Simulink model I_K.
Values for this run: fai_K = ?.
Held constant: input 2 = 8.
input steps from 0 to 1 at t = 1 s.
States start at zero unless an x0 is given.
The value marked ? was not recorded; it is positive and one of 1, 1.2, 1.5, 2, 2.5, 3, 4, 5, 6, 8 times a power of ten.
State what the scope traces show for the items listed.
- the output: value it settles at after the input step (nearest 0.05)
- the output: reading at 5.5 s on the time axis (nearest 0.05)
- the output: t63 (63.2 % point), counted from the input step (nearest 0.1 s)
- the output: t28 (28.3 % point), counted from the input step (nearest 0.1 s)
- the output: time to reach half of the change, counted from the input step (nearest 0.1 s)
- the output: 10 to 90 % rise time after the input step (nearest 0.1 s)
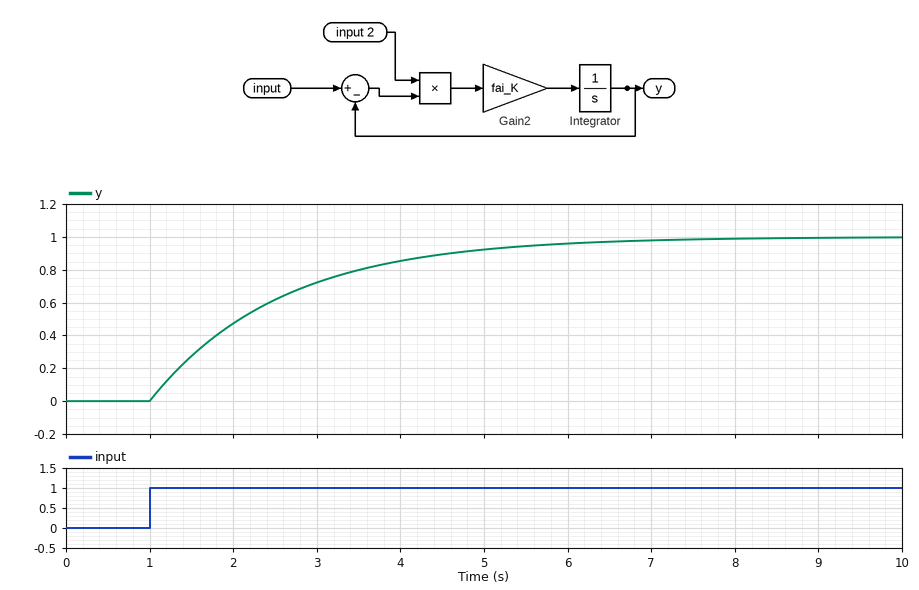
1.00
0.95
1.6 s
0.5 s
1.1 s
3.4 s
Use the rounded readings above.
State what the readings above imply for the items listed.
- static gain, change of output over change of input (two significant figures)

1.0
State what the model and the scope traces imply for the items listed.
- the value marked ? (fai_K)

0.08
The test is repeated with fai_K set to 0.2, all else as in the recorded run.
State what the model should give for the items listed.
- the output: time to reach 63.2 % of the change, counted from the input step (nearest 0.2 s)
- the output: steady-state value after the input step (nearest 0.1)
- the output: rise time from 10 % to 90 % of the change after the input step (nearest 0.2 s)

0.6 s
1.0
1.4 s
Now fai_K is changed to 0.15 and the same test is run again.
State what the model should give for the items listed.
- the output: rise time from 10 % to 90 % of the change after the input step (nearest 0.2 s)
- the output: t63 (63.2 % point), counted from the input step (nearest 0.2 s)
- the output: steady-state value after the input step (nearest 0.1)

1.8 s
0.8 s
1.0
